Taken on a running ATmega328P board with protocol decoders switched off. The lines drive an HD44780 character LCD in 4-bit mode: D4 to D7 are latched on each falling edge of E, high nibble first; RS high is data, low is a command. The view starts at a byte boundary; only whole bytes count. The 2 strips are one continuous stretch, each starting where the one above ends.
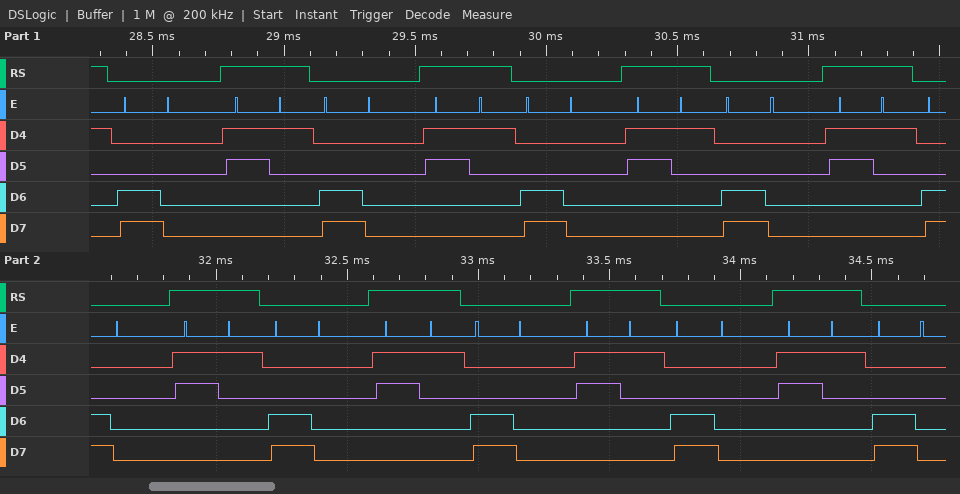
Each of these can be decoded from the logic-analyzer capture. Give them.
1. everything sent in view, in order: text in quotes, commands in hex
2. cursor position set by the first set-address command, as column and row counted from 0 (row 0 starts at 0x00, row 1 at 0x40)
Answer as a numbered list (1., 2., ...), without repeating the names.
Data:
1. 0xC0 "1" 0xC0 "1" 0xC0 "1" 0xC0 "1" 0xC0 "1" 0xC0 "1" 0xC0 "1" 0xC0 "1" 0xC0
2. column 0, row 1
